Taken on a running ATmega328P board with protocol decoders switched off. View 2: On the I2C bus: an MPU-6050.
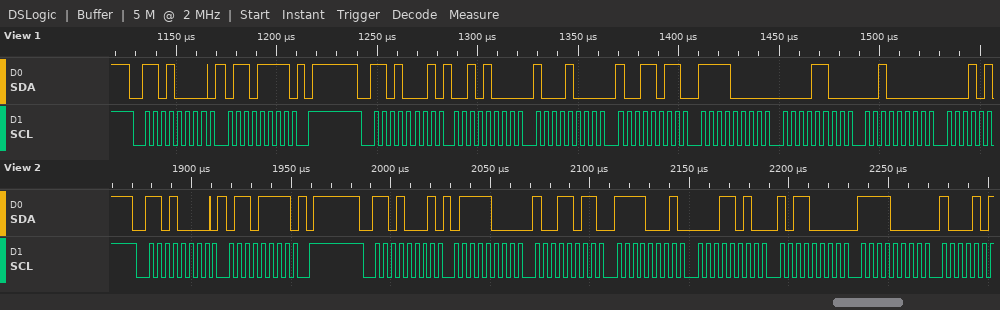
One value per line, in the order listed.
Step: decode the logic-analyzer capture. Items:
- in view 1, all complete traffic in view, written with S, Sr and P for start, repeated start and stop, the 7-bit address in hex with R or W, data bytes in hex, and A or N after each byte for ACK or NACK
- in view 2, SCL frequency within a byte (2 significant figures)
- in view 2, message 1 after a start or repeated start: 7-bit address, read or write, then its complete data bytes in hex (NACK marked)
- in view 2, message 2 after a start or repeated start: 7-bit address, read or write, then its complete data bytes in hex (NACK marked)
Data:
S 68W A 6F A P S 68R A 28 A 88 A 9B A F0 A 0C A 20 A
250 kHz
0x68 write: 6F
0x68 read: 78 9B F1 1A B0 F0
